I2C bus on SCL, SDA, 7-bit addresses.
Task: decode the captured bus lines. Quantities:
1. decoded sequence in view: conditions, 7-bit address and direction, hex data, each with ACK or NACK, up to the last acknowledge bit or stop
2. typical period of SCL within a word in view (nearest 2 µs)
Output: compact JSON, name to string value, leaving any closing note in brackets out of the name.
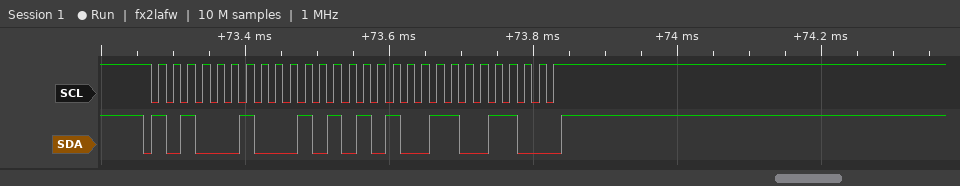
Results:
{"decoded sequence in view: conditions, 7-bit address and direction, hex data, each with ACK or NACK, up to the last acknowledge bit or stop": "start, address 51 write ACK, 55 ACK, 66 ACK, stop", "typical period of SCL within a word in view": "20 µs"}
